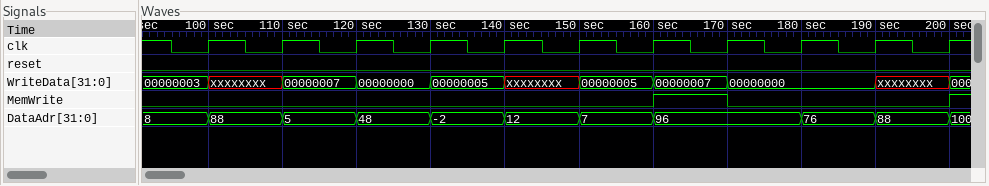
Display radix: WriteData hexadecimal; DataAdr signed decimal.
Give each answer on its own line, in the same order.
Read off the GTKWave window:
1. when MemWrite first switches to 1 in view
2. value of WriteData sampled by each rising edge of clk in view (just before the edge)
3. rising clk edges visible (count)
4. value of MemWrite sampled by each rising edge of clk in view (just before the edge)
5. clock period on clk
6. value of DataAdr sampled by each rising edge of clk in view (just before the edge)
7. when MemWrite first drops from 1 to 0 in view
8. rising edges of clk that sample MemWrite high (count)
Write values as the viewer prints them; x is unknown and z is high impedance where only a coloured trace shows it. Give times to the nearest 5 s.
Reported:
160 s
00000003, xxxxxxxx, 00000007, 00000000, 00000005, xxxxxxxx, 00000005, 00000007, 00000000, 00000000, xxxxxxxx
11
0 0 0 0 0 0 0 1 0 0 0
10 s
8, 88, 5, 48, -2, 12, 7, 96, 96, 76, 88
170 s
1
